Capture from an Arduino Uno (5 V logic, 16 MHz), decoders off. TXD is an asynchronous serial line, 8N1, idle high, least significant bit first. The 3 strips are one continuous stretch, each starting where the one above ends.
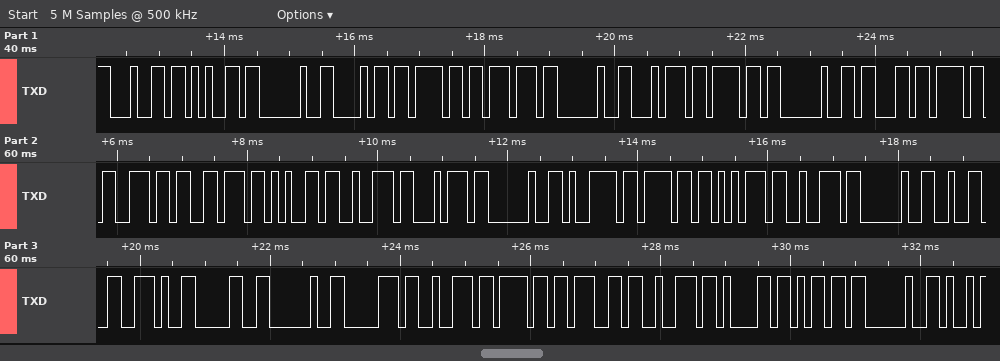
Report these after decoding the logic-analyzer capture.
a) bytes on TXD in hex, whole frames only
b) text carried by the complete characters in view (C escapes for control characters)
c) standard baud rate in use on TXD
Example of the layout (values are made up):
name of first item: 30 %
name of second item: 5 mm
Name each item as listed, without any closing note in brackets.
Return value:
bytes on TXD in hex, whole frames only: 64 65 20 68 6F 77 20 74 6F 20 63 6F 6E 76 65 72 74 20 79 6F 75 72 20 32 2E 30 20 70 72 6F 67 72 61 6D 20
text carried by the complete characters in view: "de how to convert your 2.0 program "
standard baud rate in use on TXD: 9600 baud
